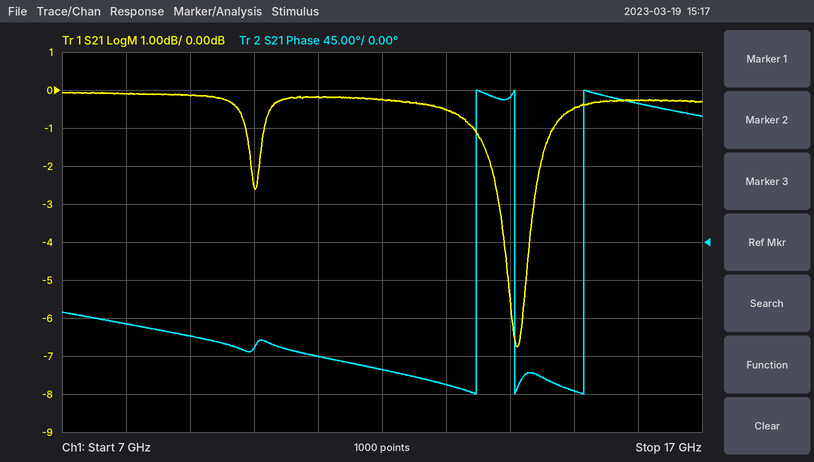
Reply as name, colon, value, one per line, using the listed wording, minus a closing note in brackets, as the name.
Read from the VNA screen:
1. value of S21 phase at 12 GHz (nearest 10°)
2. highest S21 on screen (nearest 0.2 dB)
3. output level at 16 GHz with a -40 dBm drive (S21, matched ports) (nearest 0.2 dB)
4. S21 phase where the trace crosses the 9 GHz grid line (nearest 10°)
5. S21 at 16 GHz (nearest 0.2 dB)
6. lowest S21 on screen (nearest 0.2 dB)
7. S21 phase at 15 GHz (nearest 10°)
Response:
value of S21 phase at 12 GHz: -150°
highest S21 on screen: 0.0 dB
output level at 16 GHz with a -40 dBm drive (S21, matched ports): -40.2 dBm
S21 phase where the trace crosses the 9 GHz grid line: -110°
S21 at 16 GHz: -0.2 dB
lowest S21 on screen: -6.8 dB
S21 phase at 15 GHz: -180°
